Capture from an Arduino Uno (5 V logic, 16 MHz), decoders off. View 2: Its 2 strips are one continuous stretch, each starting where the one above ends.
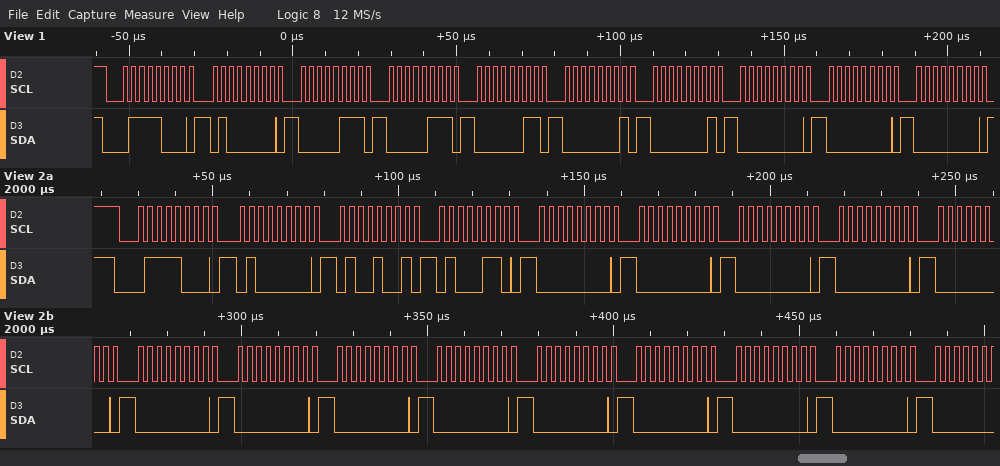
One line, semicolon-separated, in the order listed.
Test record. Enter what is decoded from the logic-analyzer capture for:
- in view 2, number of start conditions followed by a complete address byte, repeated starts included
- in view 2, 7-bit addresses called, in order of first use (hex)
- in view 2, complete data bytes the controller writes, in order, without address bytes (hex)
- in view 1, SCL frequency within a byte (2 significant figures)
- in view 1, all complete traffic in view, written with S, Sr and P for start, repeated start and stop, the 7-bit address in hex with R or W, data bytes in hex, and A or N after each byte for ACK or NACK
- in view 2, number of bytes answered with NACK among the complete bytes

1; 0x3C; 40 49 46 00 00 00 00 00 00 00 00 00 00 00 00 00; 400 kHz; S 3CW A 40 A 07 A 07 A 03 A 01 A 01 A 00 A 00 A 00 A; 0
